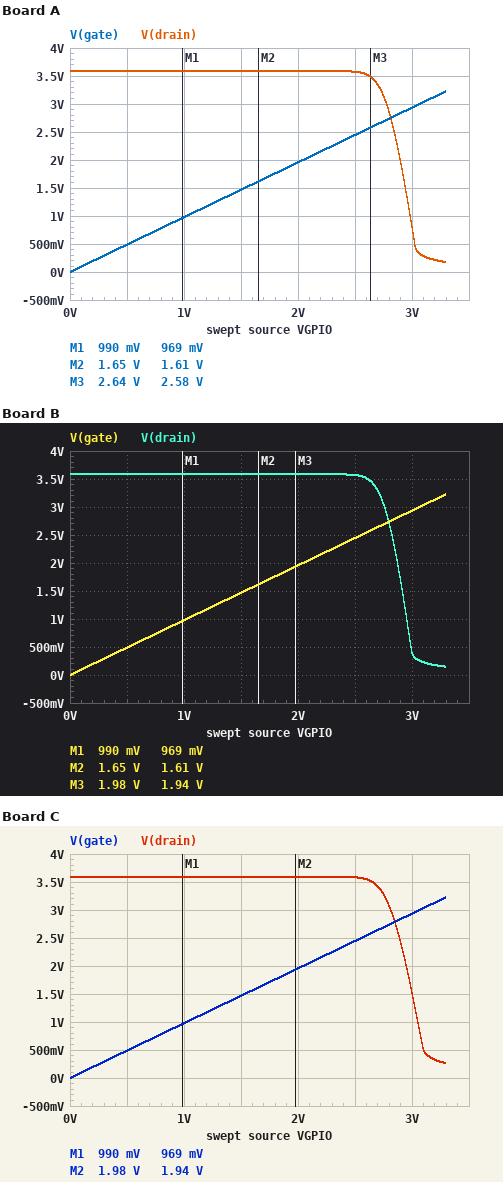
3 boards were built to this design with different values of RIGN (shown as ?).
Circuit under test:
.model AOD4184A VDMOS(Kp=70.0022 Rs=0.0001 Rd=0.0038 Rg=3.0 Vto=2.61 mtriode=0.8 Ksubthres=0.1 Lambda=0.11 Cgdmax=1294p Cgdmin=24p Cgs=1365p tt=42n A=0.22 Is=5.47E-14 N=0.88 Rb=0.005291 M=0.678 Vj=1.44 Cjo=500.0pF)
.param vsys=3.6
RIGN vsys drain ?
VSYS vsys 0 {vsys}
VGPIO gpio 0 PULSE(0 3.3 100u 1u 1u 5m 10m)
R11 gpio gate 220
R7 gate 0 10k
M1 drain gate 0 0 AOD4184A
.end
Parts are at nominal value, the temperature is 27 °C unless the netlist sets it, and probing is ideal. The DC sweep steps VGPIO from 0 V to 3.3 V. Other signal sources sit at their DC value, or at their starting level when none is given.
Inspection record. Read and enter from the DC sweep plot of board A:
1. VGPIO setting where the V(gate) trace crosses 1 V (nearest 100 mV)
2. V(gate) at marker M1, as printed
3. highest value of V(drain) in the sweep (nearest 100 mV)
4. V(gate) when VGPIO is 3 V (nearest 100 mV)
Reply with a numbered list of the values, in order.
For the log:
1. 1.0 V
2. 969 mV
3. 3.6 V
4. 2.9 V
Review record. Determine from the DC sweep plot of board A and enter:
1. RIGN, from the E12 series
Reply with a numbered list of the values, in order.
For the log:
1. 0.68 Ω
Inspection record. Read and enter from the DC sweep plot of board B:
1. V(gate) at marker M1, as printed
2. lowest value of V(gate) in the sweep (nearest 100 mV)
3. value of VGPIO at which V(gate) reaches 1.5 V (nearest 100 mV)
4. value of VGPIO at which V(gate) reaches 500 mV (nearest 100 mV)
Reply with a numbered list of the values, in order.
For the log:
1. 969 mV
2. 0 V
3. 1.5 V
4. 500 mV
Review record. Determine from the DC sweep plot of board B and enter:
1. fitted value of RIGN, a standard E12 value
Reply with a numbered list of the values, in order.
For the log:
1. 0.82 Ω
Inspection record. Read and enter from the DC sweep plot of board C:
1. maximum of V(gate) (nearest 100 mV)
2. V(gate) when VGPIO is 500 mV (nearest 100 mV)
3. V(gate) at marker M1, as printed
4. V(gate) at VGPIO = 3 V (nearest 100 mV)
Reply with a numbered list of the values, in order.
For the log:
1. 3.2 V
2. 500 mV
3. 969 mV
4. 2.9 V
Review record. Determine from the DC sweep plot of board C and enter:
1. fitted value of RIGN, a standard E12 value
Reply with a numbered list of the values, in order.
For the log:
1. 0.47 Ω
